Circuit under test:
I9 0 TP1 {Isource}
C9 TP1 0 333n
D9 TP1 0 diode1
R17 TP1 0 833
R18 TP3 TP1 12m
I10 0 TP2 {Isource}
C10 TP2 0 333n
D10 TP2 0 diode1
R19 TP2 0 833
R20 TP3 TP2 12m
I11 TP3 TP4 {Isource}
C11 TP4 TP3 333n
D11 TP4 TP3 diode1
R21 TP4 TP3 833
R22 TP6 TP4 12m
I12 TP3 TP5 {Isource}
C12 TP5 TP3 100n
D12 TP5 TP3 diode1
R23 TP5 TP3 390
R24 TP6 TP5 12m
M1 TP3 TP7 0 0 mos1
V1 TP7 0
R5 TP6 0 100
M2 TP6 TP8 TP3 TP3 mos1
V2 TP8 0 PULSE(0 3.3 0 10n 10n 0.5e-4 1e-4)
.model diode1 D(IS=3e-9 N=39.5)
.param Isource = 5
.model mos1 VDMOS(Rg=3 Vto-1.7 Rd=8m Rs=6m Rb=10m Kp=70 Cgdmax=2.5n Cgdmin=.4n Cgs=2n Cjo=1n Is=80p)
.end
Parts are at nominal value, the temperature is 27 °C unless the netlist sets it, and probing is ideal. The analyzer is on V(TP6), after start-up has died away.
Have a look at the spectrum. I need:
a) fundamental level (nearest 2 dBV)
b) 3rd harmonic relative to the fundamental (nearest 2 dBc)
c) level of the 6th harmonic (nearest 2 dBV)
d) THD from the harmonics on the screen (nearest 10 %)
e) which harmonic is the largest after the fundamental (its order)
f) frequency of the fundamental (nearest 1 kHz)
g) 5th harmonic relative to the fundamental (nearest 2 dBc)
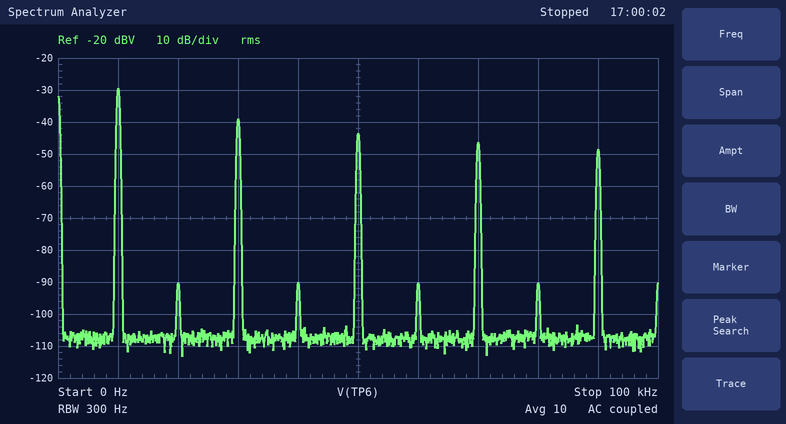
-30 dBV
-10 dBc
-90 dBV
40 %
3
10 kHz
-14 dBc
